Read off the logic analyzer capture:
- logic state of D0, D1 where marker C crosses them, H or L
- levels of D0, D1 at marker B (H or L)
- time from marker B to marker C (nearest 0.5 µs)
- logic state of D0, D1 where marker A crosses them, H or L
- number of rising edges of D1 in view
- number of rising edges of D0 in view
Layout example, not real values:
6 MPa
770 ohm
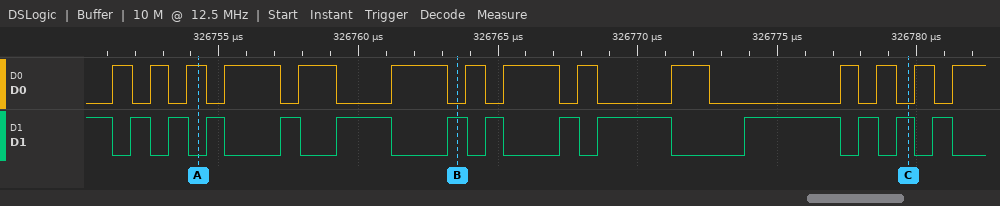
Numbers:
D0=L, D1=H
D0=L, D1=H
16 µs
D0=H, D1=L
13
14
